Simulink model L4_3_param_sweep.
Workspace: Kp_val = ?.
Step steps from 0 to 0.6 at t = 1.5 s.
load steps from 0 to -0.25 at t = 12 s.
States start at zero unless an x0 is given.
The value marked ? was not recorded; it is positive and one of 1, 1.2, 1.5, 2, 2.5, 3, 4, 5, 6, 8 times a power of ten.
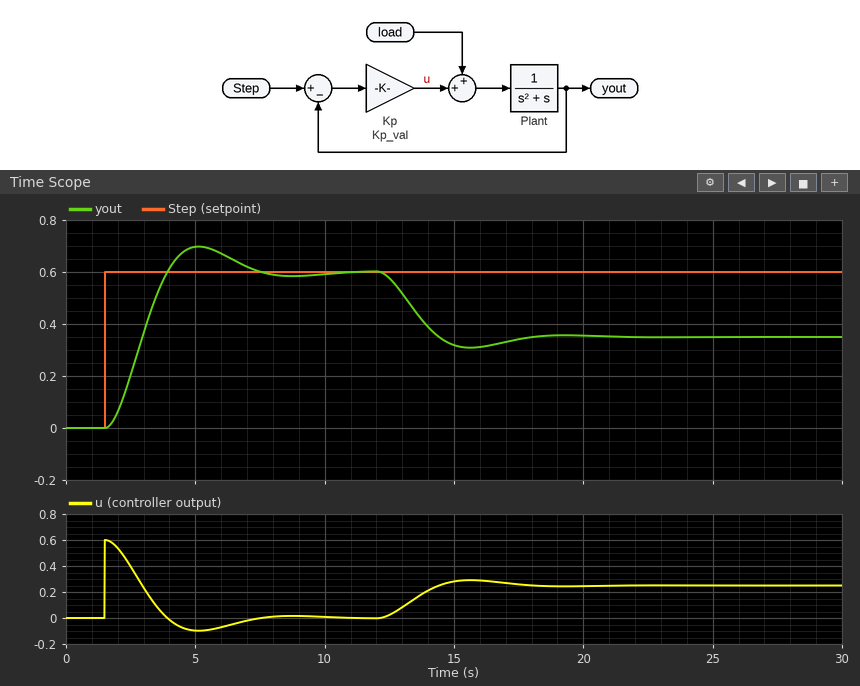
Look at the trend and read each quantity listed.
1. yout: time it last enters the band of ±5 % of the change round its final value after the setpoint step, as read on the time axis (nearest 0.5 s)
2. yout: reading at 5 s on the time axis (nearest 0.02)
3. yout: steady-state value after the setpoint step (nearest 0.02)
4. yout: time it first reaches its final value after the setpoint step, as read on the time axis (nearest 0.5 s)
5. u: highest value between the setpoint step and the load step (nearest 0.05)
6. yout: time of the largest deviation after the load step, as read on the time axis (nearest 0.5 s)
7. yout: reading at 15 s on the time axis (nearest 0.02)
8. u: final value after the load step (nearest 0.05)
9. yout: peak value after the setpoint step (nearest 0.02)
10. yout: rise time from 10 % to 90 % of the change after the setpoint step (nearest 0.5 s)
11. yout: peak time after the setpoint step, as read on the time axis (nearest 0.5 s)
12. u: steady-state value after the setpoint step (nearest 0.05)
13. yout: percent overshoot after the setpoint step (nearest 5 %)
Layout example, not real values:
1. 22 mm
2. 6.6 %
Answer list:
1. 7.0 s
2. 0.70
3. 0.60
4. 4.0 s
5. 0.60
6. 15.5 s
7. 0.32
8. 0.25
9. 0.70
10. 1.5 s
11. 5.0 s
12. 0.00
13. 15 %
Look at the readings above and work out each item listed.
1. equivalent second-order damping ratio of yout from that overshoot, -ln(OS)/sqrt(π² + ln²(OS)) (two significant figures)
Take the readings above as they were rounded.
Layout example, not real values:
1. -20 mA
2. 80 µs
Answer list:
1. 0.52
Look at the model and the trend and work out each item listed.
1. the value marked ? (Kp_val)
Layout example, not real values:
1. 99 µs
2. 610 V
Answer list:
1. 1
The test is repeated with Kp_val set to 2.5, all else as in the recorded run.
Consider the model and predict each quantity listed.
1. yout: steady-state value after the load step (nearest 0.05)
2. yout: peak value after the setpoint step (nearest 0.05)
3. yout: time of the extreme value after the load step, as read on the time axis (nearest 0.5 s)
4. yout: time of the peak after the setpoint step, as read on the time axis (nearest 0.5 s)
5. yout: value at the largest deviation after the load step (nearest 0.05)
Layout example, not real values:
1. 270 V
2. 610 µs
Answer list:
1. 0.50
2. 0.80
3. 14.0 s
4. 3.5 s
5. 0.45
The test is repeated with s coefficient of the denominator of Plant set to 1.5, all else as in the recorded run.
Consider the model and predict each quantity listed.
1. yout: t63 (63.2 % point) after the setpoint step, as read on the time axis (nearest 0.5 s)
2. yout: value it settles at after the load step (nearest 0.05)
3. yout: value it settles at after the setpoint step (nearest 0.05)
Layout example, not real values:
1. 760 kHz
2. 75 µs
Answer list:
1. 3.5 s
2. 0.35
3. 0.60
